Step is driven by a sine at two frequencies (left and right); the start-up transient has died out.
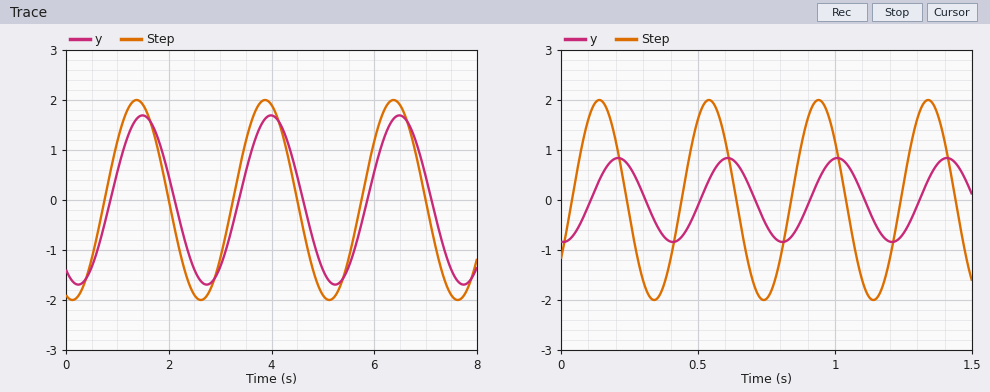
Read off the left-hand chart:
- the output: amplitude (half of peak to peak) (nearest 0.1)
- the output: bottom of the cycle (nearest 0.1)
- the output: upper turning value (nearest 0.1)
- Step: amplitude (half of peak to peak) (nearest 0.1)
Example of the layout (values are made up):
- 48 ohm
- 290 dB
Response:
- 1.7
- -1.7
- 1.7
- 2.0
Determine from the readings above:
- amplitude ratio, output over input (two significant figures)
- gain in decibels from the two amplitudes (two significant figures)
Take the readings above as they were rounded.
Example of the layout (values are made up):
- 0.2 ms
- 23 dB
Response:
- 0.85
- -1.4 dB
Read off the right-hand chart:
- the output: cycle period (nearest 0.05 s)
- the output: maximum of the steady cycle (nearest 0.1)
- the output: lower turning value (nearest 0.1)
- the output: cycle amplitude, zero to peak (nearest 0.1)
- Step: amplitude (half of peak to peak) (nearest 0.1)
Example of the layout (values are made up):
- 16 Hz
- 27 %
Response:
- 0.40 s
- 0.8
- -0.8
- 0.8
- 2.0
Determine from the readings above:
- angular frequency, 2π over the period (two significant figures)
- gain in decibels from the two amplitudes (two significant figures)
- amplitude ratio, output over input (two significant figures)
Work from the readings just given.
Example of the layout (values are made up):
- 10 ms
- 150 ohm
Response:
- 16 rad/s
- -8.0 dB
- 0.40
